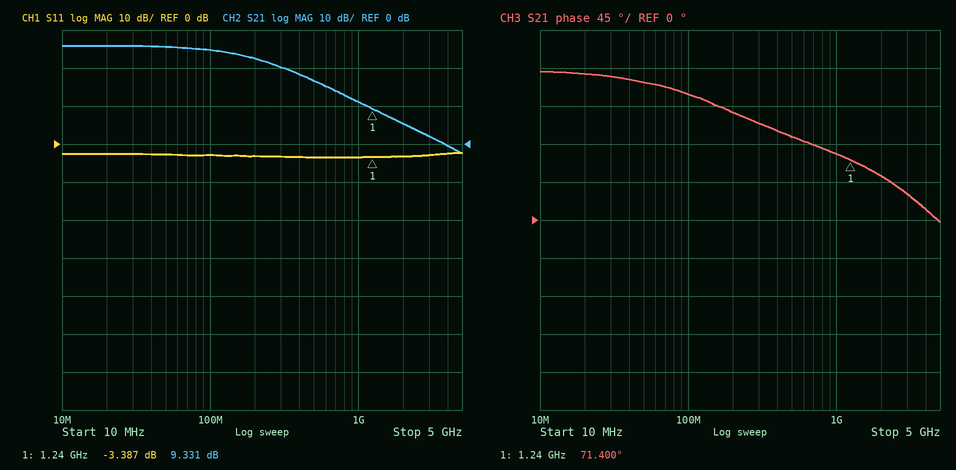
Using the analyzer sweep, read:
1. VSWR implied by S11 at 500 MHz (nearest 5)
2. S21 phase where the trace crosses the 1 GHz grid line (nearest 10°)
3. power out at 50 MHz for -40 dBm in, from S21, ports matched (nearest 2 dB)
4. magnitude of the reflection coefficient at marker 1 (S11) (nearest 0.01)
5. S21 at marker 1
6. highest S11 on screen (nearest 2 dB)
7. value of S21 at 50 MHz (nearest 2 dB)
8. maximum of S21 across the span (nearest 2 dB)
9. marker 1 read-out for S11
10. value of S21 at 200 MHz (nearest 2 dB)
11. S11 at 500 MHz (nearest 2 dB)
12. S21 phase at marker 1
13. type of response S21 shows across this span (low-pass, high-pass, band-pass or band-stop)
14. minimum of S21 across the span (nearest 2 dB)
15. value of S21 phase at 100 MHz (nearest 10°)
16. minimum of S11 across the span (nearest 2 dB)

5
80°
-14 dBm
0.68
9.331 dB
-2 dB
26 dB
26 dB
-3.387 dB
22 dB
-4 dB
71.400°
low-pass
-2 dB
150°
-4 dB
